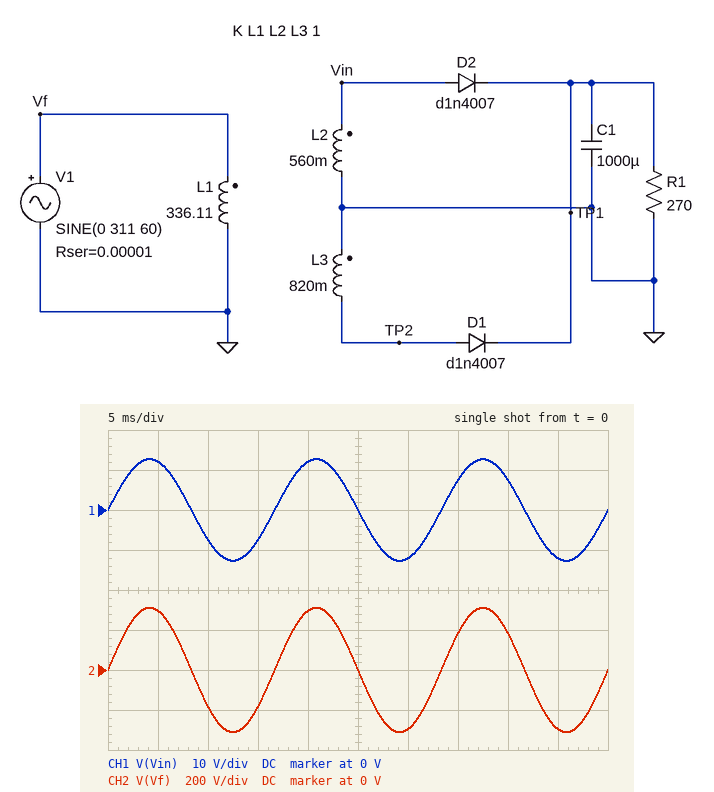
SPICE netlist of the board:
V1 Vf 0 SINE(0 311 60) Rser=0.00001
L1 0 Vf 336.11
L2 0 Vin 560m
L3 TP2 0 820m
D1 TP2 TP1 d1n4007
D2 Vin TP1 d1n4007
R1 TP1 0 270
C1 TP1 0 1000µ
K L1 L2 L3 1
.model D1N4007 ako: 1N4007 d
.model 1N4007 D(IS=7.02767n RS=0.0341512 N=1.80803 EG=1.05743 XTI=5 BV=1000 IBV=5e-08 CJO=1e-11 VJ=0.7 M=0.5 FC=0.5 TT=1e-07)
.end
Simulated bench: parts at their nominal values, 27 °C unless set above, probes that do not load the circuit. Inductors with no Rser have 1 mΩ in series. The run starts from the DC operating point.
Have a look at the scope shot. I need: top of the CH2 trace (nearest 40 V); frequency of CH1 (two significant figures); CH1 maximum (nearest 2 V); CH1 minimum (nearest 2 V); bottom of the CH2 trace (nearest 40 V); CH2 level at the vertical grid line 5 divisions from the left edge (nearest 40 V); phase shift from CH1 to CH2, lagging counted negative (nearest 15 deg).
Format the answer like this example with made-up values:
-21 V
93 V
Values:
320 V
60 Hz
12 V
-12 V
-320 V
0 V
0 deg
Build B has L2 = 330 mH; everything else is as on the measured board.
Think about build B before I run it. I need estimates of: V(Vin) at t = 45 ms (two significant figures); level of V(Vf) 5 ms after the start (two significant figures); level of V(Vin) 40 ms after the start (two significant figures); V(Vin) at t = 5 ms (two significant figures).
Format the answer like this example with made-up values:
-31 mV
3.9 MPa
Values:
-9.3 V
300 V
5.7 V
9.3 V
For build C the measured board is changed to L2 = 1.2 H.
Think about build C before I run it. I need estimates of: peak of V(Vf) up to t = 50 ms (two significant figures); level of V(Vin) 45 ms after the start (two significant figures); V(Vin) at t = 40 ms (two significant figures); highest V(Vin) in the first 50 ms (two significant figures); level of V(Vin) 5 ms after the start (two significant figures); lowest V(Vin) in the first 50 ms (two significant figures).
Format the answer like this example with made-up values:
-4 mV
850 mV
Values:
310 V
-18 V
11 V
19 V
18 V
-19 V
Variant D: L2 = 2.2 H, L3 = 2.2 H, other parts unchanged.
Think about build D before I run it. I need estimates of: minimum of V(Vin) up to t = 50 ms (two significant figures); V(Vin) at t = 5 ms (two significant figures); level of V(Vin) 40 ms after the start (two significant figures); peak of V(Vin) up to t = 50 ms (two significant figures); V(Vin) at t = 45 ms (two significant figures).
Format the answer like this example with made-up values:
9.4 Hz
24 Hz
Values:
-25 V
24 V
15 V
25 V
-24 V
